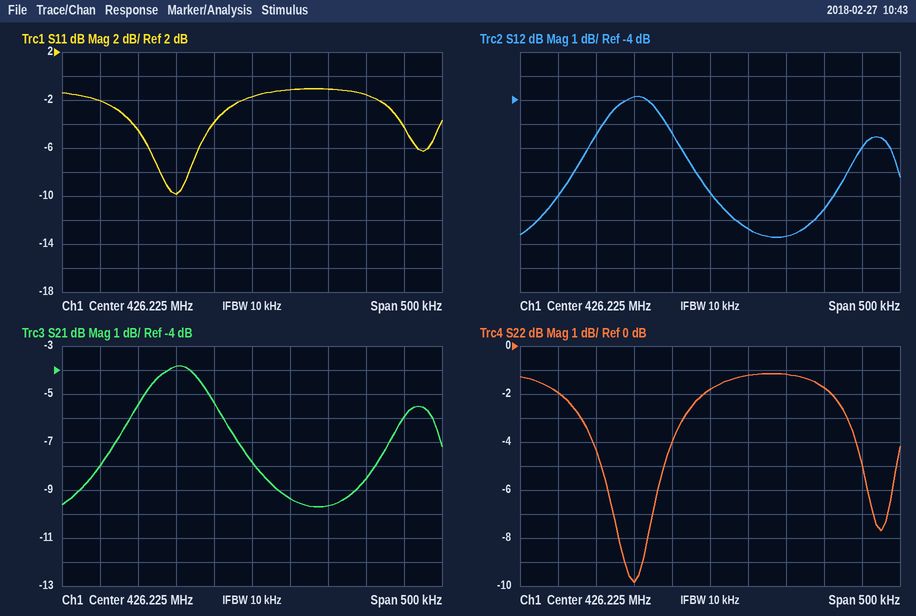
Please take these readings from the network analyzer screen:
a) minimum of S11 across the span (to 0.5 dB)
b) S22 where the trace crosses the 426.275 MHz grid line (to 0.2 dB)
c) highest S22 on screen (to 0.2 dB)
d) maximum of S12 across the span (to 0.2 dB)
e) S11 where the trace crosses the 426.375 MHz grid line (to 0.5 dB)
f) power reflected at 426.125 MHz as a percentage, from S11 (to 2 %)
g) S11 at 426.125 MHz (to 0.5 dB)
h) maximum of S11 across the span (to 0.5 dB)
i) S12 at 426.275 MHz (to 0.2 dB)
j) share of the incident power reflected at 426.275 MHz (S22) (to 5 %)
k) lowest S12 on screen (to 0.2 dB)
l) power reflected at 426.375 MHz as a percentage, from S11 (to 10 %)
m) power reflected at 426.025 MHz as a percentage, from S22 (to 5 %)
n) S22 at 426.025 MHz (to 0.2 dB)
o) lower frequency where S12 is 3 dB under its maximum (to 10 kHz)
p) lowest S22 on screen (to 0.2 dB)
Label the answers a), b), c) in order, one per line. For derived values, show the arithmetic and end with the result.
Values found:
a) -10.0 dB
b) -1.2 dB
c) -1.2 dB
d) -3.8 dB
e) -1.5 dB
f) 10^(-10/10) ≈ 10 %
g) -10.0 dB
h) -1.0 dB
i) -9.4 dB
j) 10^(-1.2/10) ≈ 75.9 %, so 75 % to the nearest 5 %
k) -9.8 dB
l) 10^(-1.5/10) ≈ 70.8 %, so 70 % to the nearest 10 %
m) 10^(-2/10) ≈ 63.1 %, so 65 % to the nearest 5 %
n) -2.0 dB
o) 426.05 MHz
p) -9.8 dB
